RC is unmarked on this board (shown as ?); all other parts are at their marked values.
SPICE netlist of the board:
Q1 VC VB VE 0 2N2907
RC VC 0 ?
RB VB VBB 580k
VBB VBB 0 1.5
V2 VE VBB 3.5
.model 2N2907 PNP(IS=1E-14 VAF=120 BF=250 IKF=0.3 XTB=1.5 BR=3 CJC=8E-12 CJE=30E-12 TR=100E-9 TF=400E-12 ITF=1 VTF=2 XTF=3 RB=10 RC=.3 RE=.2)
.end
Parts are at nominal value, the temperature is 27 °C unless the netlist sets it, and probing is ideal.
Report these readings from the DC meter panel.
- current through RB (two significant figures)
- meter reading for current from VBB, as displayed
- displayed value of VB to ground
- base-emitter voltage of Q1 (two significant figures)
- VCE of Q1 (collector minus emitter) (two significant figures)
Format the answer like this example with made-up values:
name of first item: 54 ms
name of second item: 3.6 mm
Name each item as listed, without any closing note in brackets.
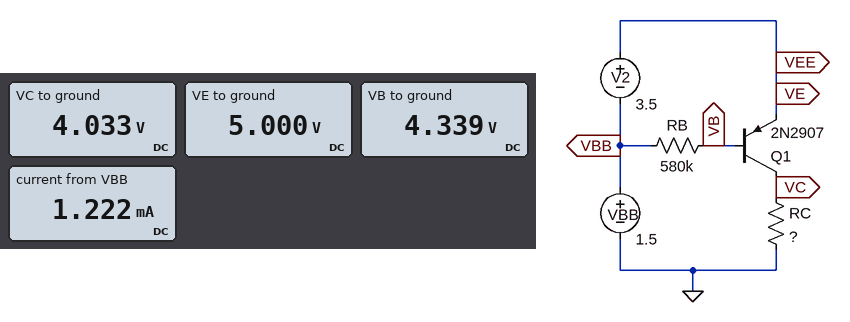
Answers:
current through RB: 4.9 µA
meter reading for current from VBB, as displayed: 1.222 mA
displayed value of VB to ground: 4.339 V
base-emitter voltage of Q1: -660 mV
VCE of Q1 (collector minus emitter): -970 mV
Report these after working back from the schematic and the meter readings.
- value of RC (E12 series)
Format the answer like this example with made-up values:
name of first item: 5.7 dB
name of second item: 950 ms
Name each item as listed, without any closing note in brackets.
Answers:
value of RC: 3.3 kΩ
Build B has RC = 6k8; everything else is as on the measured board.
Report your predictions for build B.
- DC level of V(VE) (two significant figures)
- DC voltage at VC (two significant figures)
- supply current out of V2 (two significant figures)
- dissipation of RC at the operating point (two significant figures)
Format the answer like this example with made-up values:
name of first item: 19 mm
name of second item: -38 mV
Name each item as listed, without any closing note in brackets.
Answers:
DC level of V(VE): 5.0 V
DC voltage at VC: 4.9 V
supply current out of V2: 720 µA
dissipation of RC at the operating point: 3.5 mW
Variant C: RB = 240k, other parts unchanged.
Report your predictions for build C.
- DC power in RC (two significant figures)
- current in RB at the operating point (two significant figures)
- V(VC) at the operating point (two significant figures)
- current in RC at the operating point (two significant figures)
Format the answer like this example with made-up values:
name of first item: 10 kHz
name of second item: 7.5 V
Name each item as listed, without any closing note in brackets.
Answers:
DC power in RC: 7.2 mW
current in RB at the operating point: 12 µA
V(VC) at the operating point: 4.9 V
current in RC at the operating point: 1.5 mA
